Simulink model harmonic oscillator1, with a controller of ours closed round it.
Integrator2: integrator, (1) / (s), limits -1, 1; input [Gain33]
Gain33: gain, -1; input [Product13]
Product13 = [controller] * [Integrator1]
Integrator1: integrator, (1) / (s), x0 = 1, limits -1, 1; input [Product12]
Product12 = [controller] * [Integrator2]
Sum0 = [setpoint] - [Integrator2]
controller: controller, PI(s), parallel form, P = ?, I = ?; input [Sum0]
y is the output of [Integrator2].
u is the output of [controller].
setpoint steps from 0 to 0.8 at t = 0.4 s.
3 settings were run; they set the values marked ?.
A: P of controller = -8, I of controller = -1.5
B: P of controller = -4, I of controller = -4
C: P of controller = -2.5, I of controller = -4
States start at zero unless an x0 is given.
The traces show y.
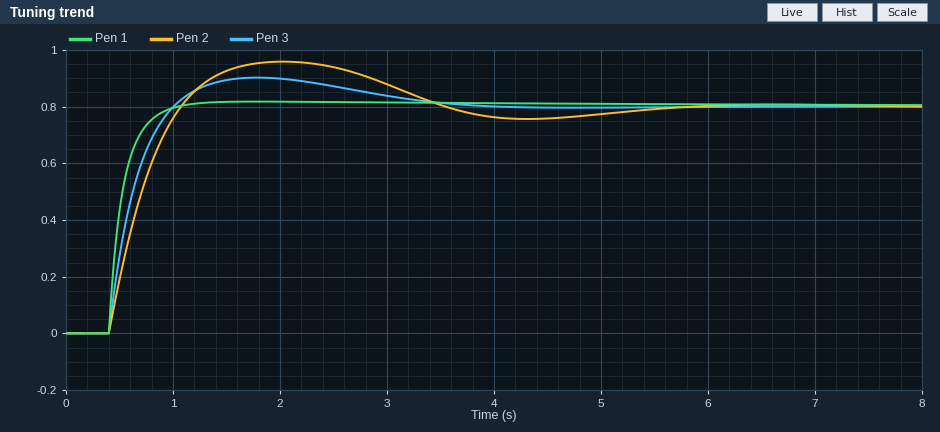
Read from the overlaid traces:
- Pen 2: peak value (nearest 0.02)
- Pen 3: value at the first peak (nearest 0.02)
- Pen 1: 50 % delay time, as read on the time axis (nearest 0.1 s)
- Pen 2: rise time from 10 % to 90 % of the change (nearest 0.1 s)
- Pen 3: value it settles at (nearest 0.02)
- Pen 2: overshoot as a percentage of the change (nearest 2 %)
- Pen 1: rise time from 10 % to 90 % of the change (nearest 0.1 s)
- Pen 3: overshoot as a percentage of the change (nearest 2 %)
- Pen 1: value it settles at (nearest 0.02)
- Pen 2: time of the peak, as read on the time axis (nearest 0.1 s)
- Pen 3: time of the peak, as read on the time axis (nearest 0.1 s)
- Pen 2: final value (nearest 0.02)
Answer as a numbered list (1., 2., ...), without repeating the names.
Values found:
1. 0.96
2. 0.90
3. 0.5 s
4. 0.5 s
5. 0.80
6. 20 %
7. 0.3 s
8. 12 %
9. 0.80
10. 2.0 s
11. 1.8 s
12. 0.80
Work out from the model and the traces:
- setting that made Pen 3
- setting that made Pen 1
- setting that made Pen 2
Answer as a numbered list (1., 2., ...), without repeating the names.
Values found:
1. B
2. A
3. C
